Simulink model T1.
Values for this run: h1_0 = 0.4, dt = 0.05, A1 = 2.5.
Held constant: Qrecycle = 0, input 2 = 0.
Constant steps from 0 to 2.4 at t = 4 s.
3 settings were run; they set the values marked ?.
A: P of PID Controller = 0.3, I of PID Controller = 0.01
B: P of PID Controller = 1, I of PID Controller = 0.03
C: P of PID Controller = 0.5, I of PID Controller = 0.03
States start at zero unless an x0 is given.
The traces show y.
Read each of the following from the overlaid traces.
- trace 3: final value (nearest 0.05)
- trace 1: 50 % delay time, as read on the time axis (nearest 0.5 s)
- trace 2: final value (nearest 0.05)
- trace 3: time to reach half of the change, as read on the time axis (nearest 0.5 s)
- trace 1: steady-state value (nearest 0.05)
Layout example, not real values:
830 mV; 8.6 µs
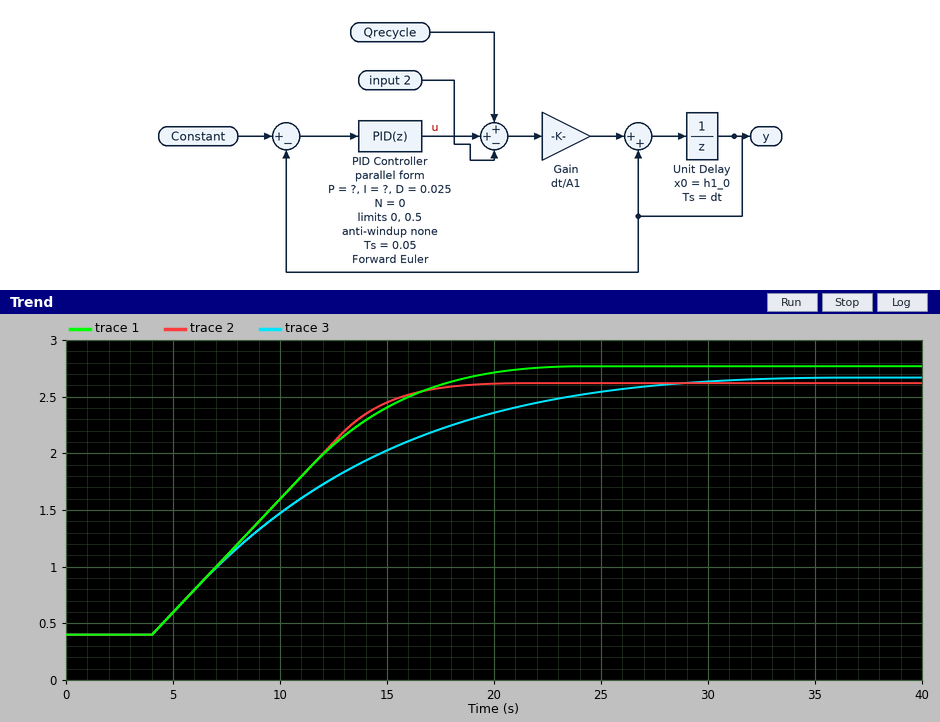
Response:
2.65; 10.0 s; 2.60; 10.5 s; 2.75
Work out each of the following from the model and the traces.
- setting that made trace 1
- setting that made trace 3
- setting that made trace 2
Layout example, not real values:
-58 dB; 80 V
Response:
C; A; B
